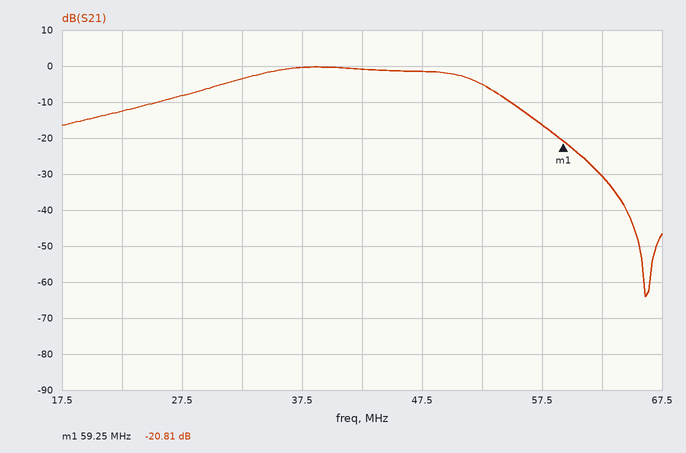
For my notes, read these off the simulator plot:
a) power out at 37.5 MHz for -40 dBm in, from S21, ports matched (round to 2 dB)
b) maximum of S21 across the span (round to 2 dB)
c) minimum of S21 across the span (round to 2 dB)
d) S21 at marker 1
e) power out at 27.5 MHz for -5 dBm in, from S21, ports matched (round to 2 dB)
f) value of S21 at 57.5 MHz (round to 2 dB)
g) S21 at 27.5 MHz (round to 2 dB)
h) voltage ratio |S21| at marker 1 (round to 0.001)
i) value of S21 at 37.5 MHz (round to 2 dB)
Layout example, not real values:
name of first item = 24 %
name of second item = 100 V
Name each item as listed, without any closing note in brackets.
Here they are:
power out at 37.5 MHz for -40 dBm in, from S21, ports matched = -40 dBm
maximum of S21 across the span = 0 dB
minimum of S21 across the span = -64 dB
S21 at marker 1 = -20.81 dB
power out at 27.5 MHz for -5 dBm in, from S21, ports matched = -14 dBm
value of S21 at 57.5 MHz = -16 dB
S21 at 27.5 MHz = -8 dB
voltage ratio |S21| at marker 1 = 0.091
value of S21 at 37.5 MHz = 0 dB
